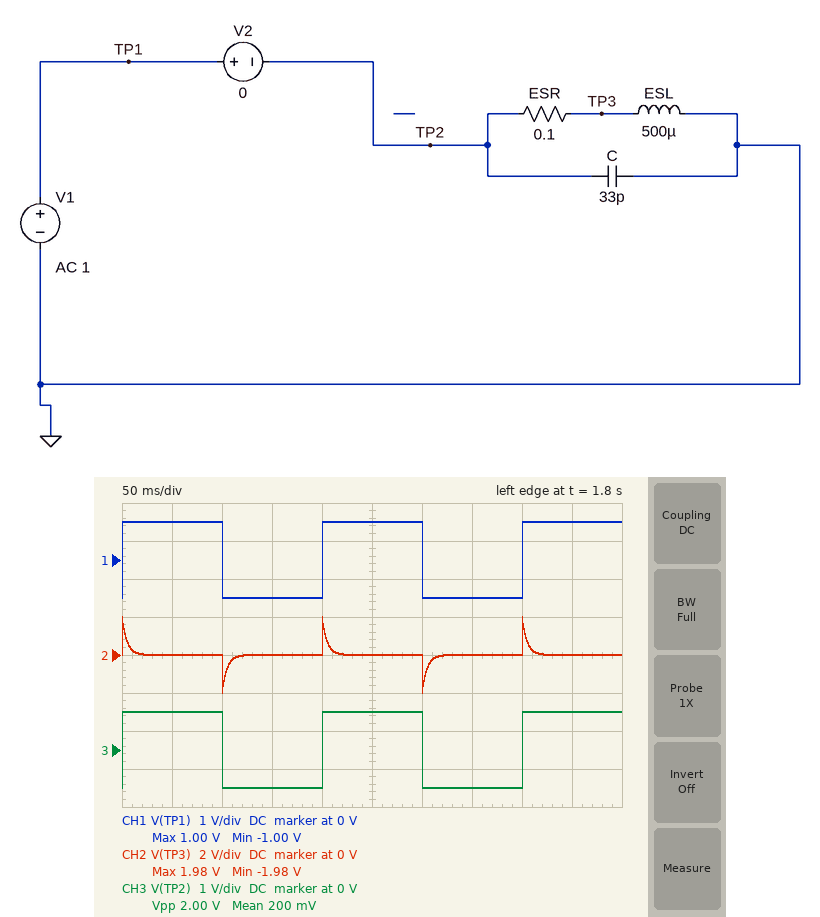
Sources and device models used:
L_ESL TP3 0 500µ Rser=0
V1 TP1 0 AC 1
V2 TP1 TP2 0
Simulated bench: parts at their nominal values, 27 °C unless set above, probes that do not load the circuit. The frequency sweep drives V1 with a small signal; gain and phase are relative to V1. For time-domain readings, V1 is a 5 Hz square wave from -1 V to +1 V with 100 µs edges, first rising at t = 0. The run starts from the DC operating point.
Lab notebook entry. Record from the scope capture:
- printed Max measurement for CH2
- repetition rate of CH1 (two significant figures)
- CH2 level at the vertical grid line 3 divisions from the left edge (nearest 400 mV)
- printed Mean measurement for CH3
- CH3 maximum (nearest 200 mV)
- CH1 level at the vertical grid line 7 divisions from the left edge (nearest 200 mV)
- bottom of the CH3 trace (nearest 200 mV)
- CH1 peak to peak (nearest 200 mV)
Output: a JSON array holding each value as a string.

["1.98 V", "5.0 Hz", "0 V", "200 mV", "1.0 V", "-1.0 V", "-1.0 V", "2.0 V"]
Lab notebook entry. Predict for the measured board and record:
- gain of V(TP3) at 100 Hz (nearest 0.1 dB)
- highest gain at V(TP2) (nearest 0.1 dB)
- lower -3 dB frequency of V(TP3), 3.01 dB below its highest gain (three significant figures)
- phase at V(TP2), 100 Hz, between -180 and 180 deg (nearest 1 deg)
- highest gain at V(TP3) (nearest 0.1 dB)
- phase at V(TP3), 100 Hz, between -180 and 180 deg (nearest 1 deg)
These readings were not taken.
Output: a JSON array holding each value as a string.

["-0.4 dB", "0 dB", "31.8 Hz", "0 deg", "0 dB", "18 deg"]
